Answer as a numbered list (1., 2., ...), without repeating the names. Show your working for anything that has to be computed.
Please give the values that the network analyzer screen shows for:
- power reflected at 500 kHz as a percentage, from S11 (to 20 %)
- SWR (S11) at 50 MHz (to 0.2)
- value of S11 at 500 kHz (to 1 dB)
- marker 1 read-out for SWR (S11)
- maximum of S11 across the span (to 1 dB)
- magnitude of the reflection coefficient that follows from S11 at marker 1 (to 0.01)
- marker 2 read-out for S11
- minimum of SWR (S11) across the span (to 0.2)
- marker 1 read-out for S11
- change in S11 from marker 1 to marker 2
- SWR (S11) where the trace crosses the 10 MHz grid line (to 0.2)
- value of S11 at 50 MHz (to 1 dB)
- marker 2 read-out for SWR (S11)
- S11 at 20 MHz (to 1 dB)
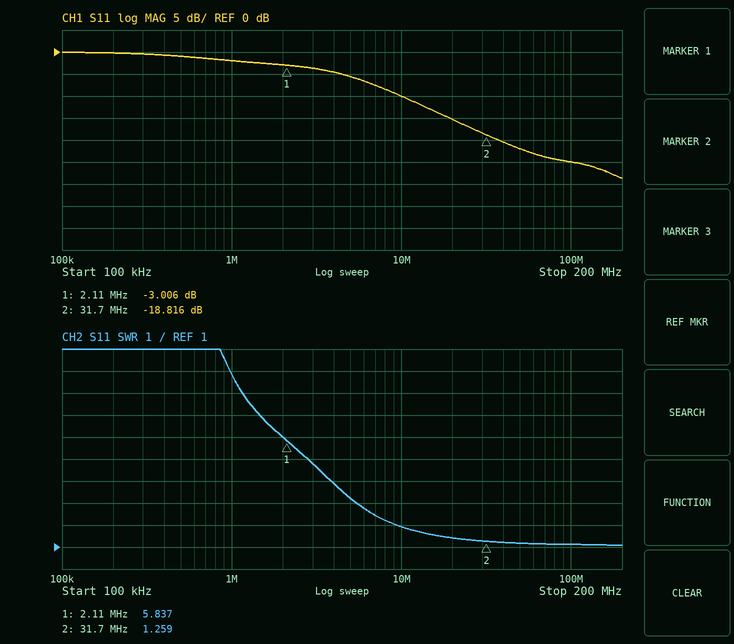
1. 10^(-1/10) ≈ 79.4 %, so 80 % to the nearest 20 %
2. 1.2
3. -1 dB
4. 5.837
5. 0 dB
6. 10^(-3.006/20) ≈ 0.71
7. -18.816 dB
8. 1.0
9. -3.006 dB
10. -18.816 − (-3.006) = -15.810 dB
11. 2.0
12. -22 dB
13. 1.259
14. -15 dB
